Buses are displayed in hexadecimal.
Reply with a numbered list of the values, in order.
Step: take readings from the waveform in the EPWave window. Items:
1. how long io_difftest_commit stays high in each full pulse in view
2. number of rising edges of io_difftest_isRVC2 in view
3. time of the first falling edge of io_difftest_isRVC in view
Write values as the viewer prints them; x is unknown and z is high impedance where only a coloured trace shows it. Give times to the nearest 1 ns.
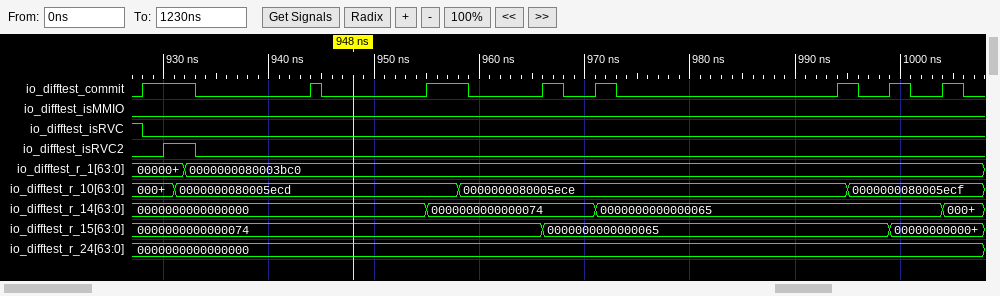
1. 5 ns, 1 ns, 4 ns, 2 ns, 2 ns, 2 ns, 2 ns, 2 ns
2. 1
3. 928 ns
